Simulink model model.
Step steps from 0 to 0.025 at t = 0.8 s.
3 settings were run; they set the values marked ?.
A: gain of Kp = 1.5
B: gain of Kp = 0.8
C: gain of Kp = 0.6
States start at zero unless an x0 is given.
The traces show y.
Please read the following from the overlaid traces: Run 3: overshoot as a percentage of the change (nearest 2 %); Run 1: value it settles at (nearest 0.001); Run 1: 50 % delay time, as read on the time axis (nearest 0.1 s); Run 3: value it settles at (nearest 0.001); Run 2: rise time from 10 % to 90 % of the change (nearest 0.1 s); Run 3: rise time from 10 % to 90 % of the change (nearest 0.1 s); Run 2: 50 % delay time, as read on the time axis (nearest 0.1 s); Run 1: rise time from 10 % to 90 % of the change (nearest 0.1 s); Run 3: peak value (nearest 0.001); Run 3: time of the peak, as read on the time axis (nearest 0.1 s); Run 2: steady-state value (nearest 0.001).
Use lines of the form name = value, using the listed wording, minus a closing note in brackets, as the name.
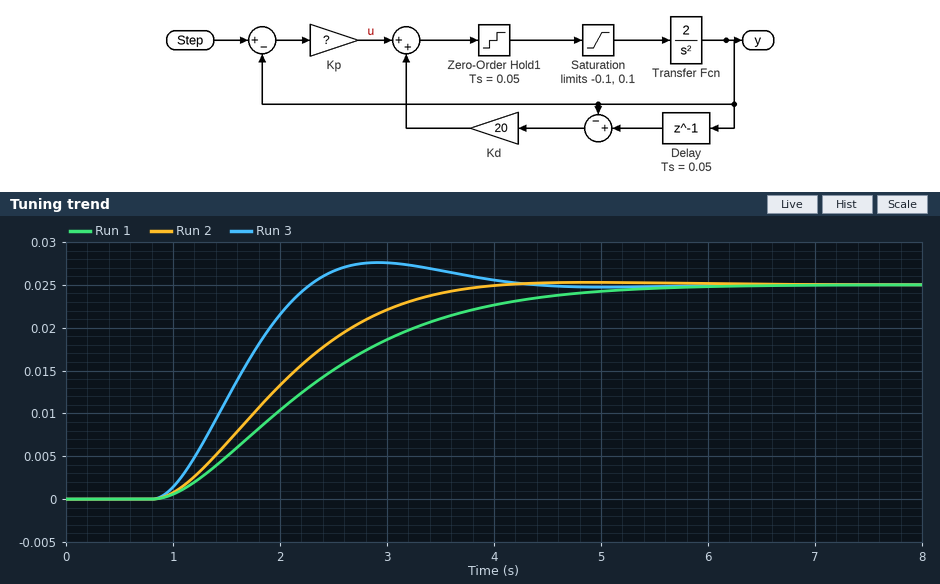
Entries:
Run 3: overshoot as a percentage of the change = 10 %
Run 1: value it settles at = 0.025
Run 1: 50 % delay time, as read on the time axis = 2.2 s
Run 3: value it settles at = 0.025
Run 2: rise time from 10 % to 90 % of the change = 1.9 s
Run 3: rise time from 10 % to 90 % of the change = 1.0 s
Run 2: 50 % delay time, as read on the time axis = 1.9 s
Run 1: rise time from 10 % to 90 % of the change = 2.7 s
Run 3: peak value = 0.028
Run 3: time of the peak, as read on the time axis = 2.9 s
Run 2: steady-state value = 0.025
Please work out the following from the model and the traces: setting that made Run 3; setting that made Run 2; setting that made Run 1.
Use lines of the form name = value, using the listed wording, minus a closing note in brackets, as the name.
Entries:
setting that made Run 3 = A
setting that made Run 2 = B
setting that made Run 1 = C
